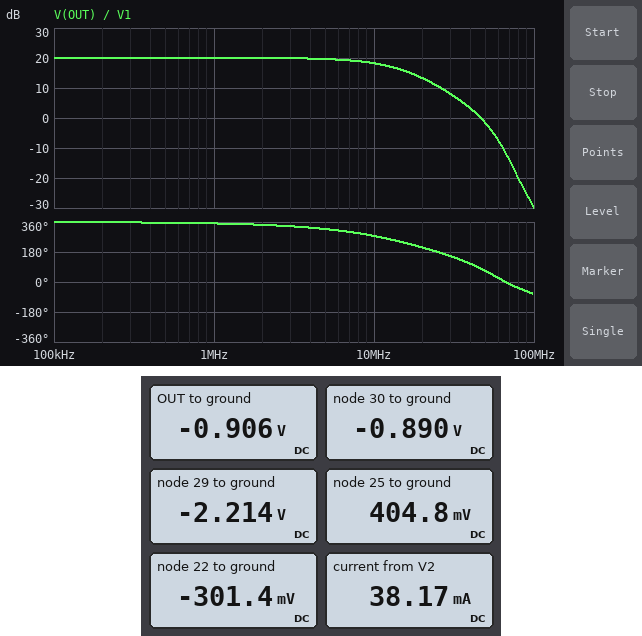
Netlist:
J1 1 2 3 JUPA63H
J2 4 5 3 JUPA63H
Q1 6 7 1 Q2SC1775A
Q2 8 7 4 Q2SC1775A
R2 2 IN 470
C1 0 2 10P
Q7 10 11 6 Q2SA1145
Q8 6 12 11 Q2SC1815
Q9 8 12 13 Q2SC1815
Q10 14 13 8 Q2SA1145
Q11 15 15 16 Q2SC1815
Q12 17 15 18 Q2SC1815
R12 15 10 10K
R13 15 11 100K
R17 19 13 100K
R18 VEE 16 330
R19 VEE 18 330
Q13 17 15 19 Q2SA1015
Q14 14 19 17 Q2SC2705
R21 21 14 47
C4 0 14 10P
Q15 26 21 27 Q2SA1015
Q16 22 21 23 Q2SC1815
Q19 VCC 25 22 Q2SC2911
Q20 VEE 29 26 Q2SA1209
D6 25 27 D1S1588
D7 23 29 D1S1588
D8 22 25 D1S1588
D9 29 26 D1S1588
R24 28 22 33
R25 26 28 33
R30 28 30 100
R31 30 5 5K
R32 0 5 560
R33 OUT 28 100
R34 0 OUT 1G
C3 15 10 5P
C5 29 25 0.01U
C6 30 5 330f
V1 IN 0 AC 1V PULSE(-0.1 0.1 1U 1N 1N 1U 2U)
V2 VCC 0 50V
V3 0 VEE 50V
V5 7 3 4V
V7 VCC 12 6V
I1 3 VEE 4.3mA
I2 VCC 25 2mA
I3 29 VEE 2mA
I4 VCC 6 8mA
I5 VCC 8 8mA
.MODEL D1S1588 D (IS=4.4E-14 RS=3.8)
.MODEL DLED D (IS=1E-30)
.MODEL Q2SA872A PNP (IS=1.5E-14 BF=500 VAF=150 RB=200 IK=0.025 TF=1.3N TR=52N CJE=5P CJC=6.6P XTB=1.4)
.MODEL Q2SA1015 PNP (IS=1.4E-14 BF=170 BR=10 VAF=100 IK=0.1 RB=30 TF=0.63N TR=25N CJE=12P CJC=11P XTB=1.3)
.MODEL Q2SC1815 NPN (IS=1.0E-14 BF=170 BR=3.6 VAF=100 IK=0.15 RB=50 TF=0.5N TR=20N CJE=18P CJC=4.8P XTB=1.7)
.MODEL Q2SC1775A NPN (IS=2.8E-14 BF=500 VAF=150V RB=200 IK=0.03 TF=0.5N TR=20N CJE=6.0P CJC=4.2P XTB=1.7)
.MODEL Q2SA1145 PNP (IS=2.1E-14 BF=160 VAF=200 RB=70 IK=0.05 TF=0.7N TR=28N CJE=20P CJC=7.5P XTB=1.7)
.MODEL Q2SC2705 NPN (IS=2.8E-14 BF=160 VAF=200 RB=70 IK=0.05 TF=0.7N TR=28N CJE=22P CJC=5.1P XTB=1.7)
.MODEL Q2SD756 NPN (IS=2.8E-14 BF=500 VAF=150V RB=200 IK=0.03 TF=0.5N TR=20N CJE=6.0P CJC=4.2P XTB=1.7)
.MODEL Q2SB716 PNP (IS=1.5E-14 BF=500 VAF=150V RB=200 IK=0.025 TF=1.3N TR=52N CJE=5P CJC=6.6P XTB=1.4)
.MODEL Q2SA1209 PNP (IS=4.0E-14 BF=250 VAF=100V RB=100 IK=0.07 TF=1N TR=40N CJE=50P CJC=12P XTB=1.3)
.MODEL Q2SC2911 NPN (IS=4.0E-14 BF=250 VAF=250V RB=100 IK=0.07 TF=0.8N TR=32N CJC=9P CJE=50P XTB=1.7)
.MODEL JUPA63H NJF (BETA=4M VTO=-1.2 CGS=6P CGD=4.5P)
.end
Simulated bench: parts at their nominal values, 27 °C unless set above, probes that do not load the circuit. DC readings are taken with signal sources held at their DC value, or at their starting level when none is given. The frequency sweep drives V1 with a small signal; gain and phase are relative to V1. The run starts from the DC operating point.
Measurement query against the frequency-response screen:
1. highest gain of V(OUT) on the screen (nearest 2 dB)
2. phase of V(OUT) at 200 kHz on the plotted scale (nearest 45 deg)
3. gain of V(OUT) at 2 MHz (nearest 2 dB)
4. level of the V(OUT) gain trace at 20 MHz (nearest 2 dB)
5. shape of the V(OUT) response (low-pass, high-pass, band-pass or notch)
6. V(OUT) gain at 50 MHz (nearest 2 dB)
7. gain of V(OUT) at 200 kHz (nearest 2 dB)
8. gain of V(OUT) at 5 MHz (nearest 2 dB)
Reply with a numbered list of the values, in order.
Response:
1. 20 dB
2. 360 deg
3. 20 dB
4. 14 dB
5. low-pass
6. -2 dB
7. 20 dB
8. 20 dB
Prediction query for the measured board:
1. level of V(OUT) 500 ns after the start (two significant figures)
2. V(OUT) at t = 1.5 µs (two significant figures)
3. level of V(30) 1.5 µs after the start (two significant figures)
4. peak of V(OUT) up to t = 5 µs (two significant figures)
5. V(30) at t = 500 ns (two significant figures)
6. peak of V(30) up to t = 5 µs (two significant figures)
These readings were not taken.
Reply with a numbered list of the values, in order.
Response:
1. -910 mV
2. 1.1 V
3. 1.1 V
4. 1.1 V
5. -890 mV
6. 1.1 V
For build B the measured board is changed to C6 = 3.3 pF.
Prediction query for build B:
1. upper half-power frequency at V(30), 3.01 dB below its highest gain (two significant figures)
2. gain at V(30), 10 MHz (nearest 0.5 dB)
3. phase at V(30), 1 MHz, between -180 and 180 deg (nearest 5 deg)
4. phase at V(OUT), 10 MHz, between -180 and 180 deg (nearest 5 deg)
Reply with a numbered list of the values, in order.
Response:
1. 5.5 MHz
2. 13.5 dB
3. -15 deg
4. -90 deg
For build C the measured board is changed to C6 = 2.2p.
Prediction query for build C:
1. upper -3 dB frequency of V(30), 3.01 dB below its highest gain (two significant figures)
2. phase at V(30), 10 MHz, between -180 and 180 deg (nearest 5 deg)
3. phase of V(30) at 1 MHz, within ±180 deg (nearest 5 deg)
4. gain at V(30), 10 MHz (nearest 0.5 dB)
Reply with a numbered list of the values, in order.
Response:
1. 7.0 MHz
2. -90 deg
3. -10 deg
4. 15.0 dB
